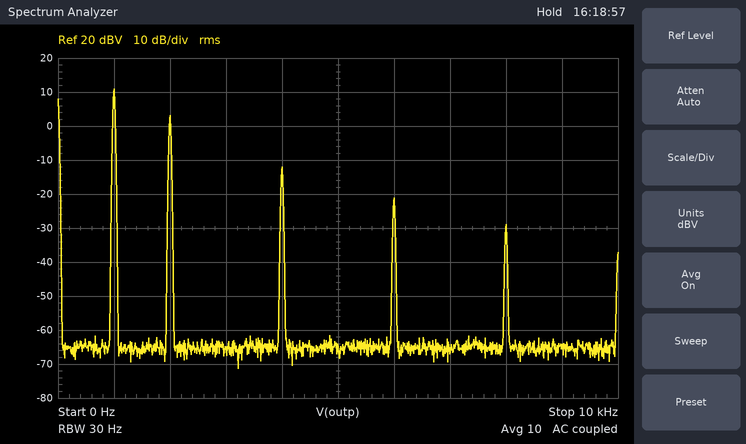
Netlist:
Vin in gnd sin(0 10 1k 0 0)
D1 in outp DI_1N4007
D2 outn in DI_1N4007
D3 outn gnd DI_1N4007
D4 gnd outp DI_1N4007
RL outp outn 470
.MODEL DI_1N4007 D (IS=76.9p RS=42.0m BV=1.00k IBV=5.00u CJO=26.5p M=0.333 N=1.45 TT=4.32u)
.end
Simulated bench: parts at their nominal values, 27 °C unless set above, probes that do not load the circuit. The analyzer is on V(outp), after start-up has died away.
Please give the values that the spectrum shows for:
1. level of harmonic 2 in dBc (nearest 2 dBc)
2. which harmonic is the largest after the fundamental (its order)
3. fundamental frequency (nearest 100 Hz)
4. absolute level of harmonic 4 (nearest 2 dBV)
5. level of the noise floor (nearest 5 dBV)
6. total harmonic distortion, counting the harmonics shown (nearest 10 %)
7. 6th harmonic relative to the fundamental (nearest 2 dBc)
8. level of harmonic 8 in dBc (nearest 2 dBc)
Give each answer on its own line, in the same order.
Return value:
-8 dBc
2
1.0 kHz
-12 dBV
-65 dBV
40 %
-32 dBc
-40 dBc
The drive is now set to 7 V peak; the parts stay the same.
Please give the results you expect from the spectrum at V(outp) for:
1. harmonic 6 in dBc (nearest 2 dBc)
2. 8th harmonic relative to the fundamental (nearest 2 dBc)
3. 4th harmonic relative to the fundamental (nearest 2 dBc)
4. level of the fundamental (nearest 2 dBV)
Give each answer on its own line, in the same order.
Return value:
-36 dBc
-50 dBc
-24 dBc
8 dBV
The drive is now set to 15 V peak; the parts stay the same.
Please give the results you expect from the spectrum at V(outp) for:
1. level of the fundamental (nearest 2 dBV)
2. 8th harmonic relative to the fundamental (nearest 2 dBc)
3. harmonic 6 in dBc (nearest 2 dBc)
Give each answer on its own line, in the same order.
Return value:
14 dBV
-36 dBc
-30 dBc
